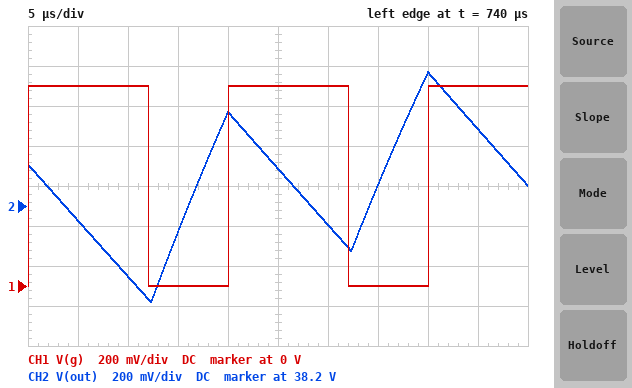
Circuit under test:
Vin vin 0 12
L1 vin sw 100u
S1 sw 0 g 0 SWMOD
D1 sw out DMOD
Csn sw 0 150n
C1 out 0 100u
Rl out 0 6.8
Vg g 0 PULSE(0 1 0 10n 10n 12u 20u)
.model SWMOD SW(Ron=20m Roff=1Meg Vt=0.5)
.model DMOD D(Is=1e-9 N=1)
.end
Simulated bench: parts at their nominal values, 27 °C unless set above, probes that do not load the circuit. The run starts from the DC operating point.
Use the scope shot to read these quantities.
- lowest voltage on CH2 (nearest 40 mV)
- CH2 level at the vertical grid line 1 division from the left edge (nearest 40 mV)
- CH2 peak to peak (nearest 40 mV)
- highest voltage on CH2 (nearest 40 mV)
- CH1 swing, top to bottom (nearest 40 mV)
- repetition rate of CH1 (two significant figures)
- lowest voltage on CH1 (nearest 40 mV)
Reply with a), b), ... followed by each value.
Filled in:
a) 37.72 V
b) 38.12 V
c) 1.16 V
d) 38.88 V
e) 1.00 V
f) 50 kHz
g) 0 V
